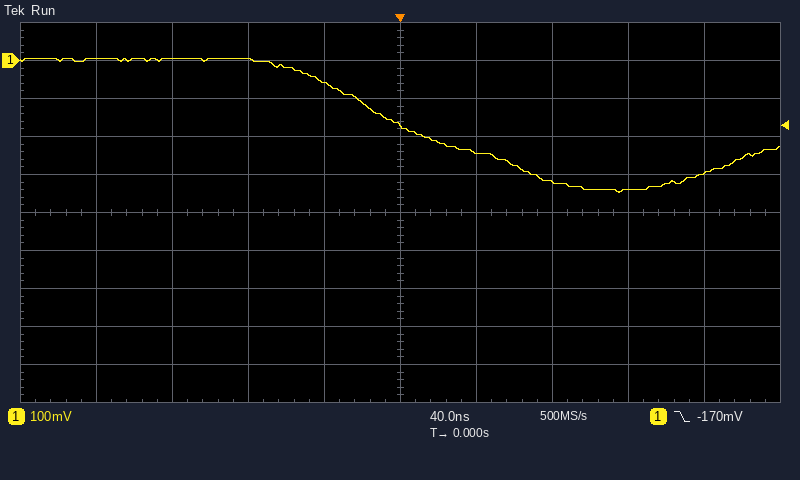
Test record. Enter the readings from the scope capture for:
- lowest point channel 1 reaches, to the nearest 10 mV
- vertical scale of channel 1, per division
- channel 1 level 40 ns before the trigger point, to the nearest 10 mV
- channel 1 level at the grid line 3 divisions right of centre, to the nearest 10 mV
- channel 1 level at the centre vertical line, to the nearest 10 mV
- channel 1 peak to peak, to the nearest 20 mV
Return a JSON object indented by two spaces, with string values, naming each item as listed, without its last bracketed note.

{
  "lowest point channel 1 reaches, to the nearest 10 mV": "-350 mV",
  "vertical scale of channel 1, per division": "100 mV",
  "channel 1 level 40 ns before the trigger point, to the nearest 10 mV": "-60 mV",
  "channel 1 level at the grid line 3 divisions right of centre, to the nearest 10 mV": "-340 mV",
  "channel 1 level at the centre vertical line, to the nearest 10 mV": "-170 mV",
  "channel 1 peak to peak, to the nearest 20 mV": "360 mV"
}
